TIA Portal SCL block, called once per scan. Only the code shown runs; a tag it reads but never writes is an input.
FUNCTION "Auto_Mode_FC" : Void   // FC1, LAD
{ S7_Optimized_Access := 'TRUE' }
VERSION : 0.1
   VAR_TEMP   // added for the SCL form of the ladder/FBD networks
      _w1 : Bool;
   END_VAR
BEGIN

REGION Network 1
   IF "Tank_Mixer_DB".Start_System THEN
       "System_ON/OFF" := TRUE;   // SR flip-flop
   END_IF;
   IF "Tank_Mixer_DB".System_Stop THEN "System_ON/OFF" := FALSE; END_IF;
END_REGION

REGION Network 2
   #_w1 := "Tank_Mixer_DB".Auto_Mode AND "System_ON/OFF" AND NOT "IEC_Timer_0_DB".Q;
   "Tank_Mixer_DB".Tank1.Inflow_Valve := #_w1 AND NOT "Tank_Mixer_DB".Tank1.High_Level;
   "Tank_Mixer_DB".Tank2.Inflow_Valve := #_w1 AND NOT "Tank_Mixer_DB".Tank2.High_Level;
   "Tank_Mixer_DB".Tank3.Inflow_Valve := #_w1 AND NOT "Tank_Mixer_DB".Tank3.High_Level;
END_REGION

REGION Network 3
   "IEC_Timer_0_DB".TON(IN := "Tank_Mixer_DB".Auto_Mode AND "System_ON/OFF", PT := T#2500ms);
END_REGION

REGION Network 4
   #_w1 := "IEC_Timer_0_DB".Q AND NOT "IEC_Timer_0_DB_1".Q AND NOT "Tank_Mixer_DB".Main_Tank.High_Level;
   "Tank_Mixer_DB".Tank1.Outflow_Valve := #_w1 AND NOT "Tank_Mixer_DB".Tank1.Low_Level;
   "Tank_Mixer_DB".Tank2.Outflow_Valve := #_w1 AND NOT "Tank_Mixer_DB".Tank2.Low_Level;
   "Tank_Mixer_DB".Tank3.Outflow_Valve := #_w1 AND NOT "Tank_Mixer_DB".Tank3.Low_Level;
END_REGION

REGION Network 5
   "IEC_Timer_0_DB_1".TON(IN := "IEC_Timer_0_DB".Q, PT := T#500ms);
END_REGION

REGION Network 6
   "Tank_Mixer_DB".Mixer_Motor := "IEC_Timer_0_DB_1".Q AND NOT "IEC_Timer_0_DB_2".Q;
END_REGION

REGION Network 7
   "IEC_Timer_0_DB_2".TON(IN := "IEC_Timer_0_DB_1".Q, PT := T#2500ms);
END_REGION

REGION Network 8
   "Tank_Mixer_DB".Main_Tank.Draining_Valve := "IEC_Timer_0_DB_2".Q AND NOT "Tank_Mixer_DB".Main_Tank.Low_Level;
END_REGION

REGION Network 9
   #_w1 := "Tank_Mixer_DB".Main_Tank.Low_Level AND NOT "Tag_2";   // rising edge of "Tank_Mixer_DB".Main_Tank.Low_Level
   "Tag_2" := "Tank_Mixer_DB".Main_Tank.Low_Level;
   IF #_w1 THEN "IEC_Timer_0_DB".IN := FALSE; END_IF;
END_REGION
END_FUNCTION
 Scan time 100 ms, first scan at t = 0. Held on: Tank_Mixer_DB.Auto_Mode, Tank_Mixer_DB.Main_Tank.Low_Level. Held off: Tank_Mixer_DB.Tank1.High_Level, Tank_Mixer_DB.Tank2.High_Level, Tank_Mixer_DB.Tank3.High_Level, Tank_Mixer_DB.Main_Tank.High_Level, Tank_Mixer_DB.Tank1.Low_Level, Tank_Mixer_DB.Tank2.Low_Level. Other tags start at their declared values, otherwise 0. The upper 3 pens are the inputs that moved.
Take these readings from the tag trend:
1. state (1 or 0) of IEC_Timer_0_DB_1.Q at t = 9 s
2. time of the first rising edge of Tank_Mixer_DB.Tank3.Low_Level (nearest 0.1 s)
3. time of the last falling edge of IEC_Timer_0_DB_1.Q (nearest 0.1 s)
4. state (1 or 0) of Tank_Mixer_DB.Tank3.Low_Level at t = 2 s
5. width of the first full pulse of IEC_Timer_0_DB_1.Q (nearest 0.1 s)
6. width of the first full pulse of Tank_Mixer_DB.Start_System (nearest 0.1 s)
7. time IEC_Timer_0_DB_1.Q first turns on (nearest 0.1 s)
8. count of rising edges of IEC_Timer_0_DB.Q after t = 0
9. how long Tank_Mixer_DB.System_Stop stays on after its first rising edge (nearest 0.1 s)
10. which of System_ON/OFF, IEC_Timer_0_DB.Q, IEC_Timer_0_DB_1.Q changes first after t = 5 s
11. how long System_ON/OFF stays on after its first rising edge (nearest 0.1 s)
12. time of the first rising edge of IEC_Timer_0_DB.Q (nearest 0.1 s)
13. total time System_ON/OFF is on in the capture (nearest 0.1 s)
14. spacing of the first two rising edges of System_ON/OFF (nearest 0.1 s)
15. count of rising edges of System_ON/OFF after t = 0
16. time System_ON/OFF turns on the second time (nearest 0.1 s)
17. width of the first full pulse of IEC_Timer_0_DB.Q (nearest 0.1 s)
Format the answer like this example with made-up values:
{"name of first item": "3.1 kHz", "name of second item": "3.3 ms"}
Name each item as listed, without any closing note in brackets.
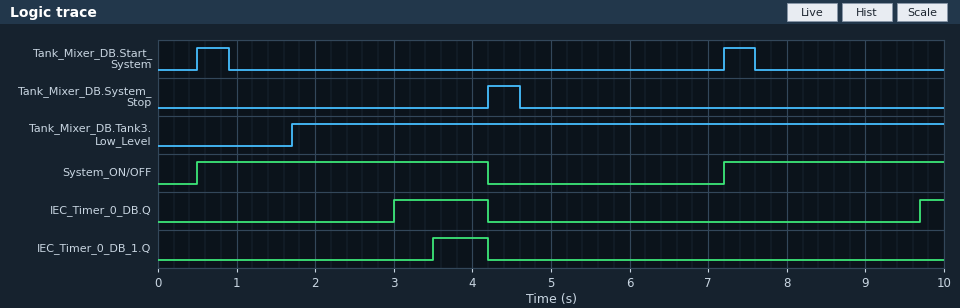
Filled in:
{"state (1 or 0) of IEC_Timer_0_DB_1.Q at t = 9 s": "0", "time of the first rising edge of Tank_Mixer_DB.Tank3.Low_Level": "1.7 s", "time of the last falling edge of IEC_Timer_0_DB_1.Q": "4.2 s", "state (1 or 0) of Tank_Mixer_DB.Tank3.Low_Level at t = 2 s": "1", "width of the first full pulse of IEC_Timer_0_DB_1.Q": "0.7 s", "width of the first full pulse of Tank_Mixer_DB.Start_System": "0.4 s", "time IEC_Timer_0_DB_1.Q first turns on": "3.5 s", "count of rising edges of IEC_Timer_0_DB.Q after t = 0": "2", "how long Tank_Mixer_DB.System_Stop stays on after its first rising edge": "0.4 s", "which of System_ON/OFF, IEC_Timer_0_DB.Q, IEC_Timer_0_DB_1.Q changes first after t = 5 s": "System_ON/OFF", "how long System_ON/OFF stays on after its first rising edge": "3.7 s", "time of the first rising edge of IEC_Timer_0_DB.Q": "3.0 s", "total time System_ON/OFF is on in the capture": "6.5 s", "spacing of the first two rising edges of System_ON/OFF": "6.7 s", "count of rising edges of System_ON/OFF after t = 0": "2", "time System_ON/OFF turns on the second time": "7.2 s", "width of the first full pulse of IEC_Timer_0_DB.Q": "1.2 s"}
